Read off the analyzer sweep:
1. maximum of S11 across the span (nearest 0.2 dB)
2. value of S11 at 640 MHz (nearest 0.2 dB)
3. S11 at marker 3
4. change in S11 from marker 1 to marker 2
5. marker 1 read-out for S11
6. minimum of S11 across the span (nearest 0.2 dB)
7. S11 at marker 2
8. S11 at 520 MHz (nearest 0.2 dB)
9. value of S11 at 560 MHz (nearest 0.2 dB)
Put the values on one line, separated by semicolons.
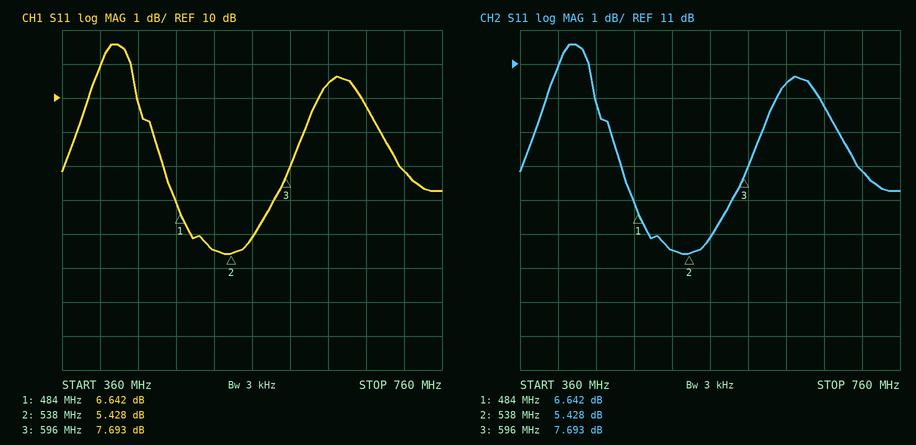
11.6 dB; 10.4 dB; 7.693 dB; -1.214 dB; 6.642 dB; 5.4 dB; 5.428 dB; 5.6 dB; 5.8 dB
